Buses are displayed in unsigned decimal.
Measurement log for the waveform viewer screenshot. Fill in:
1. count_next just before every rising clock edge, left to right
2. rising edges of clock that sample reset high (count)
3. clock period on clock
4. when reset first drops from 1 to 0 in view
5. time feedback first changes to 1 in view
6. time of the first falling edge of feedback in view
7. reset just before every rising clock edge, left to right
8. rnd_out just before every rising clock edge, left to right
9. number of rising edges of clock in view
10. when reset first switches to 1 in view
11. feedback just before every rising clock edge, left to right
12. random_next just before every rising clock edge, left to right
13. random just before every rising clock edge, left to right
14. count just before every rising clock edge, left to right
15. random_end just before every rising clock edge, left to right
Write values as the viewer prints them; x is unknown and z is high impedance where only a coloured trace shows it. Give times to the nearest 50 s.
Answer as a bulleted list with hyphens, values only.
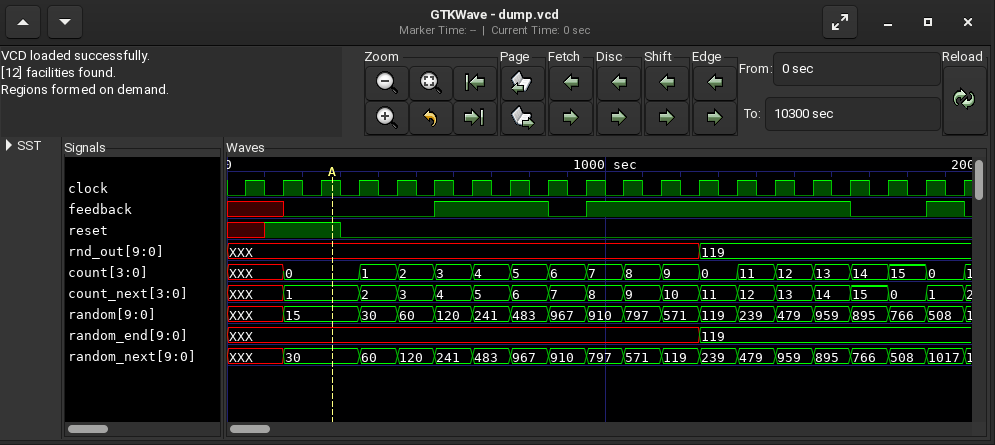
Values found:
- XXX, XXX, 1, 1, 2, 3, 4, 5, 6, 7, 8, 9, 10, 11, 12, 13, 14, 15, 0, 1
- 2
- 100 s
- 300 s
- 550 s
- 850 s
- x 1 1 0 0 0 0 0 0 0 0 0 0 0 0 0 0 0 0 0
- XXX, XXX, XXX, XXX, XXX, XXX, XXX, XXX, XXX, XXX, XXX, XXX, XXX, 119, 119, 119, 119, 119, 119, 119
- 20
- 100 s
- x x 0 0 0 0 1 1 1 0 1 1 1 1 1 1 1 0 0 1
- XXX, XXX, 30, 30, 60, 120, 241, 483, 967, 910, 797, 571, 119, 239, 479, 959, 895, 766, 508, 1017
- XXX, XXX, 15, 15, 30, 60, 120, 241, 483, 967, 910, 797, 571, 119, 239, 479, 959, 895, 766, 508
- XXX, XXX, 0, 0, 1, 2, 3, 4, 5, 6, 7, 8, 9, 0, 11, 12, 13, 14, 15, 0
- XXX, XXX, XXX, XXX, XXX, XXX, XXX, XXX, XXX, XXX, XXX, XXX, XXX, 119, 119, 119, 119, 119, 119, 119
